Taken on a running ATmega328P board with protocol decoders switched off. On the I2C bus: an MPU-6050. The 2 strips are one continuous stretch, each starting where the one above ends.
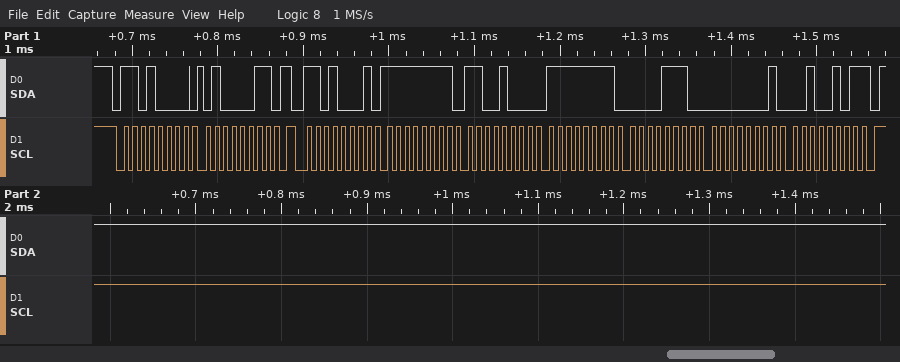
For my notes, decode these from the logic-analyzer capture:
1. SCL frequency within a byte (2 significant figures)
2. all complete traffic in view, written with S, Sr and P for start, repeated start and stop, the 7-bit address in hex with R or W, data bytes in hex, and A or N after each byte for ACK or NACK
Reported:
100 kHz
S 68W A 43 A Sr 68R A FF A C8 A FF A 0E A 01 A 25 N P
